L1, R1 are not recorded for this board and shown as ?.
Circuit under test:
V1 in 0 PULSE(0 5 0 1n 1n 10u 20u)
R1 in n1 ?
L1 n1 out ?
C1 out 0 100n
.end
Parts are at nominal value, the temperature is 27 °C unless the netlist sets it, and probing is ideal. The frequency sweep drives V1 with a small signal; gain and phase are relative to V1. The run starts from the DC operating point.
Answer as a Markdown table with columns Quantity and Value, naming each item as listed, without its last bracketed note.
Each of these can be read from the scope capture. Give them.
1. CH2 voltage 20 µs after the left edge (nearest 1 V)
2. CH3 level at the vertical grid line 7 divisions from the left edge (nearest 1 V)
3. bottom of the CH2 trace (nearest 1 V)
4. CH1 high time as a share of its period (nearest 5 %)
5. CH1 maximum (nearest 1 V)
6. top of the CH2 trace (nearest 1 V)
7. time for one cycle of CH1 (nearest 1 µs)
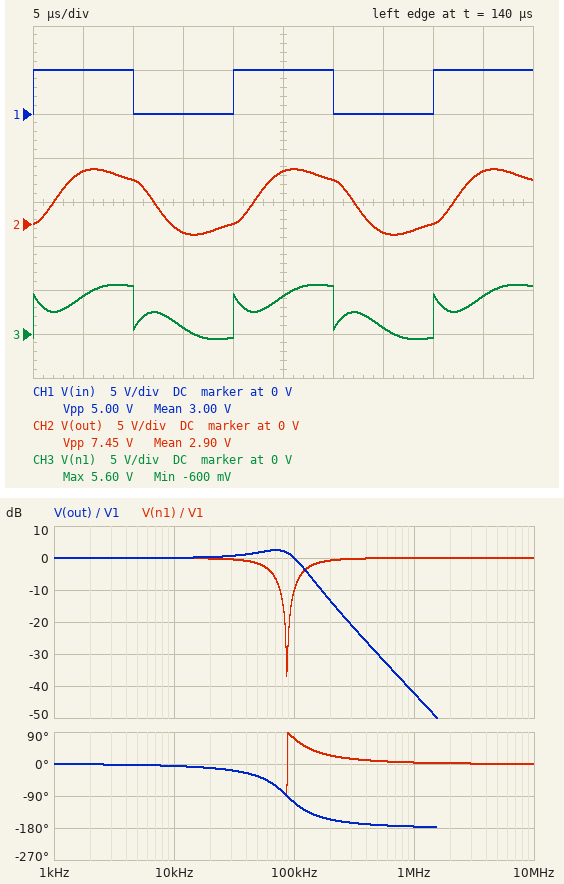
| Quantity | Value |
|---|---|
| CH2 voltage 20 µs after the left edge | 0 V |
| CH3 level at the vertical grid line 7 divisions from the left edge | 1 V |
| bottom of the CH2 trace | -1 V |
| CH1 high time as a share of its period | 50 % |
| CH1 maximum | 5 V |
| top of the CH2 trace | 6 V |
| time for one cycle of CH1 | 20 µs |
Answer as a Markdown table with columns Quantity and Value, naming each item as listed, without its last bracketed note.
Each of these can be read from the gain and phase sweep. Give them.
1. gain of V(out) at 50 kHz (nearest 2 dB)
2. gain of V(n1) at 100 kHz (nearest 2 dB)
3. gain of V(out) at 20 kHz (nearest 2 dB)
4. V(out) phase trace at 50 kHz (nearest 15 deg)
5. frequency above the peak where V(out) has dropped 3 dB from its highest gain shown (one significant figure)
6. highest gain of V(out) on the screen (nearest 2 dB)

| Quantity | Value |
|---|---|
| gain of V(out) at 50 kHz | 2 dB |
| gain of V(n1) at 100 kHz | -10 dB |
| gain of V(out) at 20 kHz | 0 dB |
| V(out) phase trace at 50 kHz | -30 deg |
| frequency above the peak where V(out) has dropped 3 dB from its highest gain shown | 100 kHz |
| highest gain of V(out) on the screen | 2 dB |
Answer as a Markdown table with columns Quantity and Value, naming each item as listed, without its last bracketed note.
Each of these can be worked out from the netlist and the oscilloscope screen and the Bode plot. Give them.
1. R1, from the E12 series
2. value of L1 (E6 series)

| Quantity | Value |
|---|---|
| R1, from the E12 series | 15 Ω |
| value of L1 | 33 µH |
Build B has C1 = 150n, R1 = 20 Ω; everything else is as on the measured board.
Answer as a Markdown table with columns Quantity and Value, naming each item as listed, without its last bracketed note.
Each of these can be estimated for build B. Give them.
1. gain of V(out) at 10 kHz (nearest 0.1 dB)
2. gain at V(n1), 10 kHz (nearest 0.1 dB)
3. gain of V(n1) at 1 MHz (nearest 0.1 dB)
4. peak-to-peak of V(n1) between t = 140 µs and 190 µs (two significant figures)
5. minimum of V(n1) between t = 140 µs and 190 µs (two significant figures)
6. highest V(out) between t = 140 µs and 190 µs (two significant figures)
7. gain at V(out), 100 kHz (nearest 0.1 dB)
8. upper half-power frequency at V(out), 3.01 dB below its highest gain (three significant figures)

| Quantity | Value |
|---|---|
| gain of V(out) at 10 kHz | 0 dB |
| gain at V(n1), 10 kHz | -0.2 dB |
| gain of V(n1) at 1 MHz | 0 dB |
| peak-to-peak of V(n1) between t = 140 µs and 190 µs | 5.2 V |
| minimum of V(n1) between t = 140 µs and 190 µs | -86 mV |
| highest V(out) between t = 140 µs and 190 µs | 5.3 V |
| gain at V(out), 100 kHz | -6.5 dB |
| upper half-power frequency at V(out), 3.01 dB below its highest gain | 74.6 kHz |
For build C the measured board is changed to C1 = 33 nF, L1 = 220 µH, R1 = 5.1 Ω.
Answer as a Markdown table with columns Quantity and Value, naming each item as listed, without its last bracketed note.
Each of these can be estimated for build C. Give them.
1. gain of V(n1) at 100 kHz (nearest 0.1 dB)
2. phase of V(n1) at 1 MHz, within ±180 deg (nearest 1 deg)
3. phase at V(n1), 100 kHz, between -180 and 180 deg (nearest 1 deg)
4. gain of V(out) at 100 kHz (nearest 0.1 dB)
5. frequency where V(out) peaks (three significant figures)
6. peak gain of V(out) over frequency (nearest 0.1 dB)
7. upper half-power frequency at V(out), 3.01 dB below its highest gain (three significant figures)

| Quantity | Value |
|---|---|
| gain of V(n1) at 100 kHz | 0 dB |
| phase of V(n1) at 1 MHz, within ±180 deg | 0 deg |
| phase at V(n1), 100 kHz, between -180 and 180 deg | 3 deg |
| gain of V(out) at 100 kHz | -5.4 dB |
| frequency where V(out) peaks | 59.0 kHz |
| peak gain of V(out) over frequency | 24.1 dB |
| upper half-power frequency at V(out), 3.01 dB below its highest gain | 60.8 kHz |
